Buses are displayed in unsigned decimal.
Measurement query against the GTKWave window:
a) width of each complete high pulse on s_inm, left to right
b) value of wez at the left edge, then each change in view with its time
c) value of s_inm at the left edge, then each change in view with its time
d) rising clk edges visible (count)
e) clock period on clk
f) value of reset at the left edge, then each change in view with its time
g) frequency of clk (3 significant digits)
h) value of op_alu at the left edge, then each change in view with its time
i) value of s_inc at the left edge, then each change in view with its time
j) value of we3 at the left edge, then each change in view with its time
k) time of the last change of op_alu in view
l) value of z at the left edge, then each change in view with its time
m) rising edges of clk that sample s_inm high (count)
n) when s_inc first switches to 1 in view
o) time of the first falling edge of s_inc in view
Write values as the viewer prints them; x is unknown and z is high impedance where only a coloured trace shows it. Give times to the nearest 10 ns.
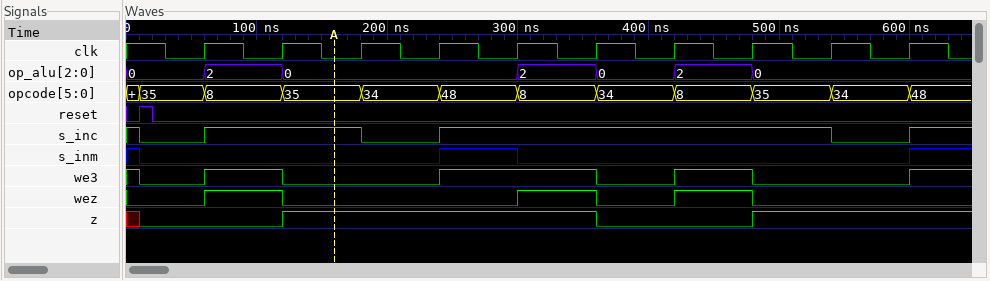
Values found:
60 ns
0, 1 at 60 ns, 0 at 120 ns, 1 at 300 ns, 0 at 360 ns, 1 at 420 ns, 0 at 480 ns
1, 0 at 10 ns, 1 at 240 ns, 0 at 300 ns, 1 at 600 ns
10
60 ns
0, 1 at 10 ns, 0 at 20 ns
16.7 MHz
0, 2 at 60 ns, 0 at 120 ns, 2 at 300 ns, 0 at 360 ns, 2 at 420 ns, 0 at 480 ns
1, 0 at 10 ns, 1 at 60 ns, 0 at 180 ns, 1 at 240 ns, 0 at 540 ns, 1 at 600 ns
1, 0 at 10 ns, 1 at 60 ns, 0 at 120 ns, 1 at 240 ns, 0 at 360 ns, 1 at 420 ns, 0 at 480 ns, 1 at 600 ns
480 ns
x, 0 at 10 ns, 1 at 120 ns, 0 at 360 ns, 1 at 480 ns
1
60 ns
10 ns
